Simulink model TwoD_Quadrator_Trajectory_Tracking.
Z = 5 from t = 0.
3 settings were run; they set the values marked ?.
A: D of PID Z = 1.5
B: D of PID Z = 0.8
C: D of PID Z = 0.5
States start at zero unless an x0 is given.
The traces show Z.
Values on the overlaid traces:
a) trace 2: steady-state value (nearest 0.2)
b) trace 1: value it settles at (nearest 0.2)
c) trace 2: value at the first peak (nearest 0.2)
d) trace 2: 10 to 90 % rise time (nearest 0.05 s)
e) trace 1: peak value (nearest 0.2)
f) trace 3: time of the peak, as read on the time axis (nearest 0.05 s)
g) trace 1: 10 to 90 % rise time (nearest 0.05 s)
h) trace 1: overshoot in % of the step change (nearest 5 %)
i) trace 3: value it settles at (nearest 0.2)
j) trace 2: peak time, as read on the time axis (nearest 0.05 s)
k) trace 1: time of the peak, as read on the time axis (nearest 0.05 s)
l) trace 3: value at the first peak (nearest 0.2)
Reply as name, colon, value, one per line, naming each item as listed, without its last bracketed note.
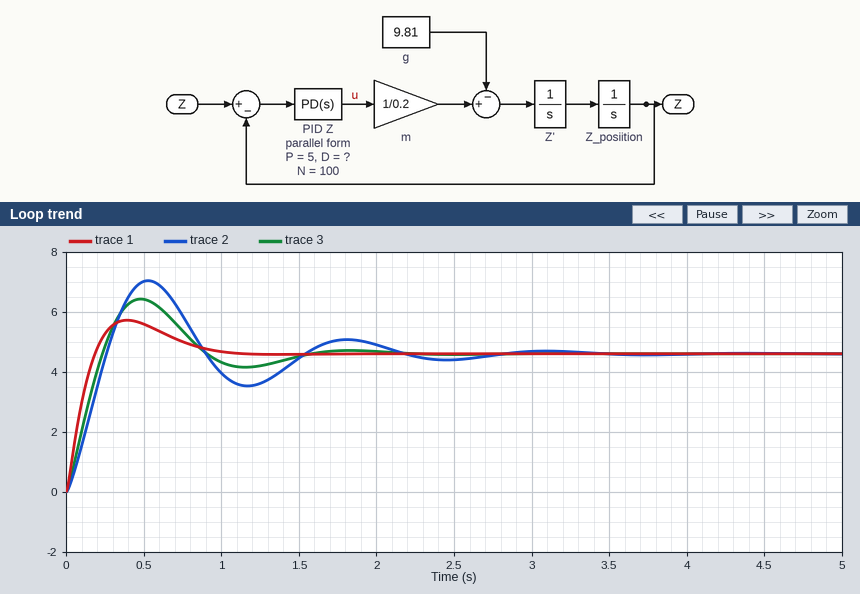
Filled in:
trace 2: steady-state value: 4.6
trace 1: value it settles at: 4.6
trace 2: value at the first peak: 7.0
trace 2: 10 to 90 % rise time: 0.20 s
trace 1: peak value: 5.8
trace 3: time of the peak, as read on the time axis: 0.50 s
trace 1: 10 to 90 % rise time: 0.15 s
trace 1: overshoot in % of the step change: 25 %
trace 3: value it settles at: 4.6
trace 2: peak time, as read on the time axis: 0.55 s
trace 1: time of the peak, as read on the time axis: 0.40 s
trace 3: value at the first peak: 6.4
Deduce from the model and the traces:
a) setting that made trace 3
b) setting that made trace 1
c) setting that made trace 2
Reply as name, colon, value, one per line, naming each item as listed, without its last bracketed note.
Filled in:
setting that made trace 3: B
setting that made trace 1: A
setting that made trace 2: C
